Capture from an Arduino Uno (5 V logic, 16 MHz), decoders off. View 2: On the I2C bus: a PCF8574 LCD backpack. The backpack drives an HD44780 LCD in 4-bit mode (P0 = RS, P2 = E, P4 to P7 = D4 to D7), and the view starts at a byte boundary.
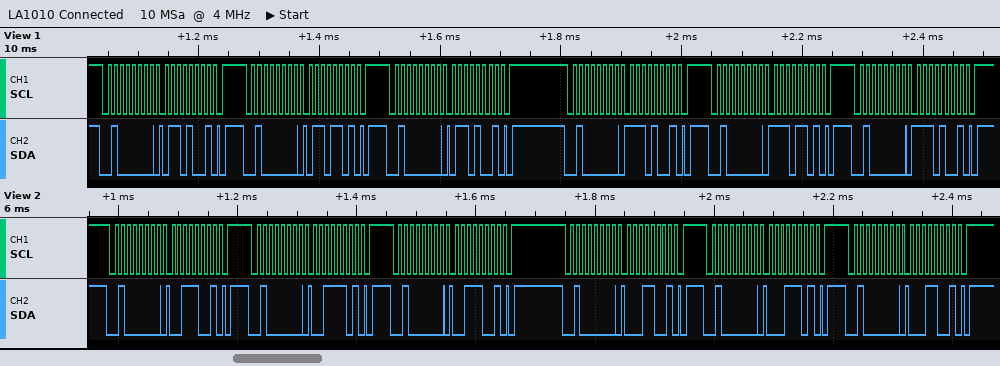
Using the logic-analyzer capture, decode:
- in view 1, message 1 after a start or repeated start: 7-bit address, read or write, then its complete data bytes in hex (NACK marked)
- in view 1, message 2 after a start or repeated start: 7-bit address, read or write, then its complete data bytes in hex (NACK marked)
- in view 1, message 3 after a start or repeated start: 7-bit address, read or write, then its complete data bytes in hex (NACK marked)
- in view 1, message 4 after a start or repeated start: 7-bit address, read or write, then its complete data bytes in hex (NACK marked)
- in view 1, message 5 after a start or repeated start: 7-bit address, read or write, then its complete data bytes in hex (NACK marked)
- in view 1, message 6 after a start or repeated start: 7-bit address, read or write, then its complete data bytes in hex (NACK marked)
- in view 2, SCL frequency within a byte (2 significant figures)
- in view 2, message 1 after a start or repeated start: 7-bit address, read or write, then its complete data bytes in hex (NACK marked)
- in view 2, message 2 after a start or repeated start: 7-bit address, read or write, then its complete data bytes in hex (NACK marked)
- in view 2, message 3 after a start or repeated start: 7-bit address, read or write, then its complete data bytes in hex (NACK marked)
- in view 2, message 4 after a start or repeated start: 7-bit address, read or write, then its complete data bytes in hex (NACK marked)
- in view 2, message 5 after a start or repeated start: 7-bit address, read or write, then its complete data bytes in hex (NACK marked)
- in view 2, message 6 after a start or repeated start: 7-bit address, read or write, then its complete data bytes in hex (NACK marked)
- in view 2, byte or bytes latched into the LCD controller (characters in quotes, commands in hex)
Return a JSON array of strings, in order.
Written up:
["0x20 write: 69", "0x20 write: 6D", "0x20 write: 69", "0x20 write: E9", "0x20 write: ED", "0x20 write: E9", "100 kHz", "0x20 write: 39", "0x20 write: 3D", "0x20 write: 39", "0x20 write: 19", "0x20 write: 1D", "0x20 write: 19", "'1'"]
